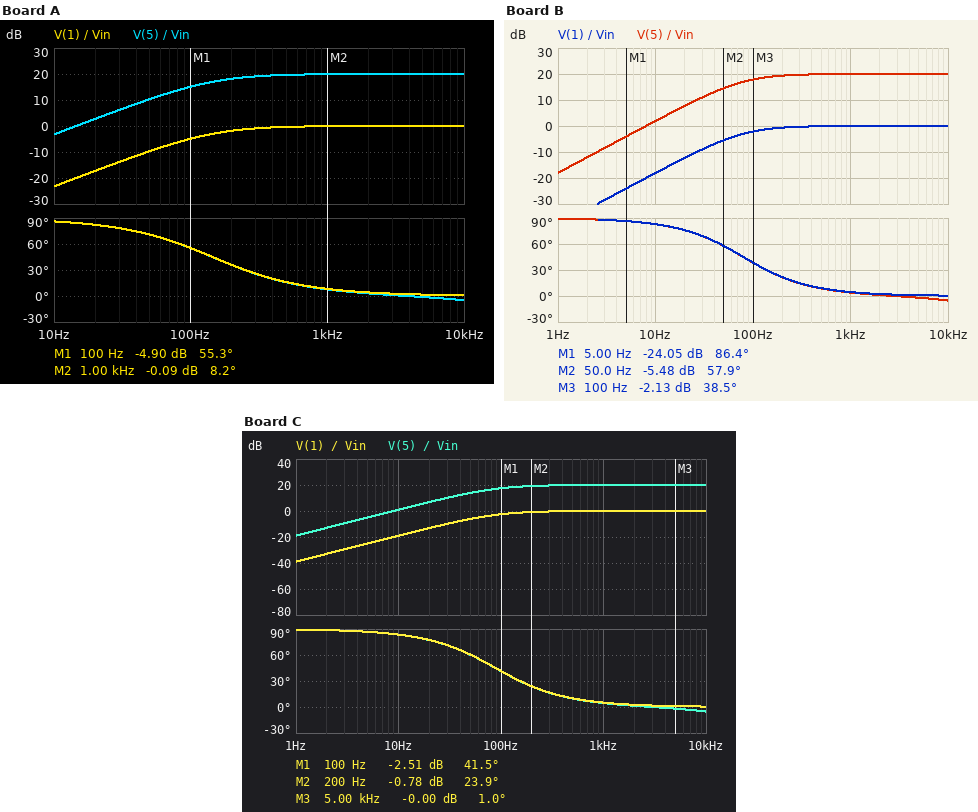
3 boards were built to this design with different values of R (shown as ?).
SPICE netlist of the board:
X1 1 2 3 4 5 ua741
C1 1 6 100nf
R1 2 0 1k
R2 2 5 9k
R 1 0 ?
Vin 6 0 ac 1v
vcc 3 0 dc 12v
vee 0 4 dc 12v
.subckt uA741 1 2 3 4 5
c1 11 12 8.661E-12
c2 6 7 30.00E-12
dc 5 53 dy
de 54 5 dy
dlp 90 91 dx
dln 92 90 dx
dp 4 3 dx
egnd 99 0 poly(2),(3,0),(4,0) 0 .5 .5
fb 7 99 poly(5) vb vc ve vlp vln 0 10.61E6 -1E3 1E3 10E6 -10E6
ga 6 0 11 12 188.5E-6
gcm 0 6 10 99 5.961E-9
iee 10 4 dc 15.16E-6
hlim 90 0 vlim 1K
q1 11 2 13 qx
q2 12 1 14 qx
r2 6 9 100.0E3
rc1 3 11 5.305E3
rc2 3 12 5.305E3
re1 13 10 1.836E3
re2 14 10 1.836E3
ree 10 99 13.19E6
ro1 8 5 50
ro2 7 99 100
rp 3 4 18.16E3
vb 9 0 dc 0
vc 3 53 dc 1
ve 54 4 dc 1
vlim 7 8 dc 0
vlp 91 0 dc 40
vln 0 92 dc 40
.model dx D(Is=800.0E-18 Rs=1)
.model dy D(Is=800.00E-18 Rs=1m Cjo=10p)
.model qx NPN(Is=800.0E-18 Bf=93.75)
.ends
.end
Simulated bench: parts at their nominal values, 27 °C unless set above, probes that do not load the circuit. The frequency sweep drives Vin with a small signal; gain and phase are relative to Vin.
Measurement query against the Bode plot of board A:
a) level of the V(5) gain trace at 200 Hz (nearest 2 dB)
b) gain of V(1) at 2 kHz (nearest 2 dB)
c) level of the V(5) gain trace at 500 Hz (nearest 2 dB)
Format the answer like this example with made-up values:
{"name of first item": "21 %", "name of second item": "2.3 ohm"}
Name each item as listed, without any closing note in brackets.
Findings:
{"level of the V(5) gain trace at 200 Hz": "18 dB", "gain of V(1) at 2 kHz": "0 dB", "level of the V(5) gain trace at 500 Hz": "20 dB"}
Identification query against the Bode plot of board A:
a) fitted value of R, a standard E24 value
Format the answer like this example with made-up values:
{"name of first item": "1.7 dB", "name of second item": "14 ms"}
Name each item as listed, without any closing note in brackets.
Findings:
{"fitted value of R, a standard E24 value": "11 kΩ"}
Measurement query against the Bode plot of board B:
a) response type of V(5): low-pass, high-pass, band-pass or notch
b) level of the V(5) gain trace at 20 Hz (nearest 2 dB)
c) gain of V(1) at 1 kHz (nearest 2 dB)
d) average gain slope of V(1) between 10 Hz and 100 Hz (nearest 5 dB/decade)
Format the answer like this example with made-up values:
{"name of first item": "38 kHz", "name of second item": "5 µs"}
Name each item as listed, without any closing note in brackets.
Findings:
{"response type of V(5): low-pass, high-pass, band-pass or notch": "high-pass", "level of the V(5) gain trace at 20 Hz": "8 dB", "gain of V(1) at 1 kHz": "0 dB", "average gain slope of V(1) between 10 Hz and 100 Hz": "15 dB/decade"}
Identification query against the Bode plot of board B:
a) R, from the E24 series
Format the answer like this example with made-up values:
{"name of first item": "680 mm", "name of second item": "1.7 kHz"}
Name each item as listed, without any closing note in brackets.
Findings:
{"R, from the E24 series": "20 kΩ"}
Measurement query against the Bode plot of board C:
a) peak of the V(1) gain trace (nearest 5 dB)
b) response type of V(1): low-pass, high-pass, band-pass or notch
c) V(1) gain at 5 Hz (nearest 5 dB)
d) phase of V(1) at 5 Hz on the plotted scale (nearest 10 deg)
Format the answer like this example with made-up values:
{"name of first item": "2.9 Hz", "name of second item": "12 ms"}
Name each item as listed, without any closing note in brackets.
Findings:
{"peak of the V(1) gain trace": "0 dB", "response type of V(1): low-pass, high-pass, band-pass or notch": "high-pass", "V(1) gain at 5 Hz": "-25 dB", "phase of V(1) at 5 Hz on the plotted scale": "90 deg"}
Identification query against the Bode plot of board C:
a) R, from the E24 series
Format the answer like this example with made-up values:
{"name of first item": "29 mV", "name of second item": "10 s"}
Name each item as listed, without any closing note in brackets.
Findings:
{"R, from the E24 series": "18 kΩ"}
